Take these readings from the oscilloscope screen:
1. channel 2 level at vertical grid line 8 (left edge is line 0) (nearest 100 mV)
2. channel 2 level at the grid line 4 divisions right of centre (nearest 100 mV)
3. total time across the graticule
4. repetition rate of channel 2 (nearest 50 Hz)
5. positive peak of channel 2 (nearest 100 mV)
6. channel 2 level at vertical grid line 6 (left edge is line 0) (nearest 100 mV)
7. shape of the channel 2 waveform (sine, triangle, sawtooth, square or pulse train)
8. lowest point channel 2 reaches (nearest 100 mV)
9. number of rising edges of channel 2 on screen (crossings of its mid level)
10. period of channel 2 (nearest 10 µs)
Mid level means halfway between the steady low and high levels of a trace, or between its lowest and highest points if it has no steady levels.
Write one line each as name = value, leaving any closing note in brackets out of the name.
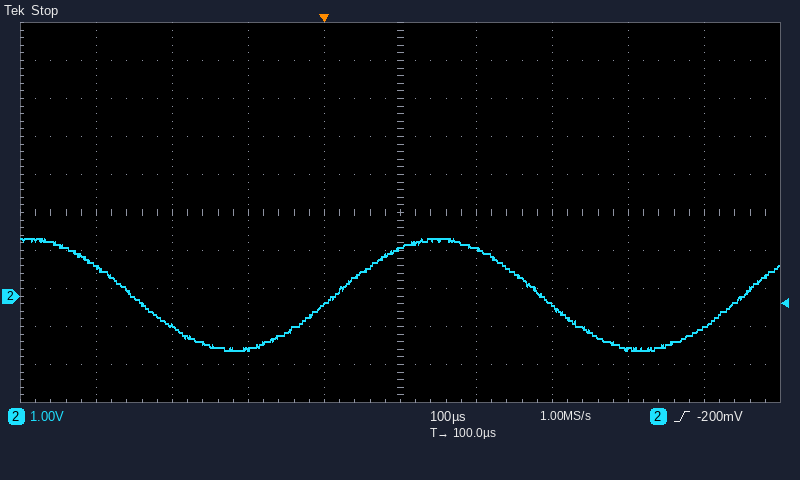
channel 2 level at vertical grid line 8 (left edge is line 0) = -1.4 V
channel 2 level at the grid line 4 divisions right of centre = -800 mV
total time across the graticule = 1 ms
repetition rate of channel 2 = 1.85 kHz
positive peak of channel 2 = 1.5 V
channel 2 level at vertical grid line 6 (left edge is line 0) = 1.2 V
shape of the channel 2 waveform = sine
lowest point channel 2 reaches = -1.4 V
number of rising edges of channel 2 on screen = 2
period of channel 2 = 540 µs
